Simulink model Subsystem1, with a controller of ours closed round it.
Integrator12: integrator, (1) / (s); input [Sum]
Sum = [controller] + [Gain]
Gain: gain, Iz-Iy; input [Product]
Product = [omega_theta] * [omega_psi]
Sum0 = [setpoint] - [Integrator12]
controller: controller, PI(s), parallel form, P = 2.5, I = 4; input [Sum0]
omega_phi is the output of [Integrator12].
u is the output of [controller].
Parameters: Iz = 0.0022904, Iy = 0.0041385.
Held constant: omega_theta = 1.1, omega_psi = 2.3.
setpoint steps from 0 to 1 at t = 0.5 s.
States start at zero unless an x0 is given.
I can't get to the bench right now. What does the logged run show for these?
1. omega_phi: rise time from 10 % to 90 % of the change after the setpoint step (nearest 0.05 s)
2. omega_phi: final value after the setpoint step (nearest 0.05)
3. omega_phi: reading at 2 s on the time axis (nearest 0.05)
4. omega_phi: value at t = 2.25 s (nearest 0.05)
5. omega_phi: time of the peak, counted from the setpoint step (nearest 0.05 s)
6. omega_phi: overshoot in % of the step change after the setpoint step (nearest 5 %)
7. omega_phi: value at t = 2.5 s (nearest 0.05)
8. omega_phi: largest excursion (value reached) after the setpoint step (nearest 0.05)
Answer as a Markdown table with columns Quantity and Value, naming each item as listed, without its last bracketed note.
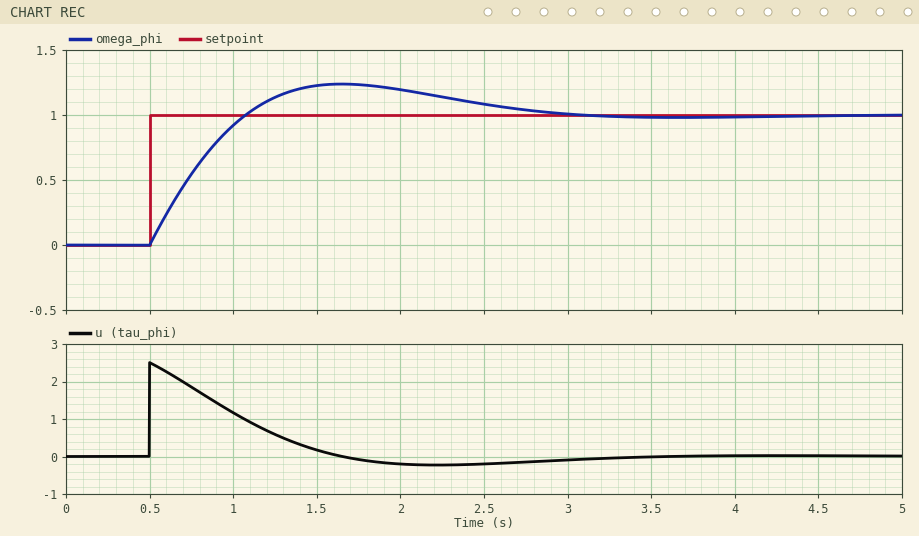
| Quantity | Value |
|---|---|
| omega_phi: rise time from 10 % to 90 % of the change after the setpoint step | 0.45 s |
| omega_phi: final value after the setpoint step | 1.00 |
| omega_phi: reading at 2 s on the time axis | 1.20 |
| omega_phi: value at t = 2.25 s | 1.15 |
| omega_phi: time of the peak, counted from the setpoint step | 1.15 s |
| omega_phi: overshoot in % of the step change after the setpoint step | 25 % |
| omega_phi: value at t = 2.5 s | 1.10 |
| omega_phi: largest excursion (value reached) after the setpoint step | 1.25 |
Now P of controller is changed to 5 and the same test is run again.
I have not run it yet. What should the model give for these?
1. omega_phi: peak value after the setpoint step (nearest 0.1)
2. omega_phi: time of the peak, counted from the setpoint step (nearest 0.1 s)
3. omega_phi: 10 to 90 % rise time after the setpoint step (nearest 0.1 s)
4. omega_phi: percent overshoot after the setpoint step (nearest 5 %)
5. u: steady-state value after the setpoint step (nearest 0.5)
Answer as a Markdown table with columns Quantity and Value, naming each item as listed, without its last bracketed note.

| Quantity | Value |
|---|---|
| omega_phi: peak value after the setpoint step | 1.1 |
| omega_phi: time of the peak, counted from the setpoint step | 0.9 s |
| omega_phi: 10 to 90 % rise time after the setpoint step | 0.3 s |
| omega_phi: percent overshoot after the setpoint step | 10 % |
| u: steady-state value after the setpoint step | 0.0 |
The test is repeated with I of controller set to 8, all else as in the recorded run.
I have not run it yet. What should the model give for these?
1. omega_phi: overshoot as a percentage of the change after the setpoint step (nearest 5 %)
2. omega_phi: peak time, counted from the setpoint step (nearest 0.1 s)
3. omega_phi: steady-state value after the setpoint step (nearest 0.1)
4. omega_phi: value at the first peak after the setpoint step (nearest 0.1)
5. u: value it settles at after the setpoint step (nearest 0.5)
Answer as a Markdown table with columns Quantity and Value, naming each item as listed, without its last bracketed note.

| Quantity | Value |
|---|---|
| omega_phi: overshoot as a percentage of the change after the setpoint step | 35 % |
| omega_phi: peak time, counted from the setpoint step | 0.9 s |
| omega_phi: steady-state value after the setpoint step | 1.0 |
| omega_phi: value at the first peak after the setpoint step | 1.3 |
| u: value it settles at after the setpoint step | 0.0 |
